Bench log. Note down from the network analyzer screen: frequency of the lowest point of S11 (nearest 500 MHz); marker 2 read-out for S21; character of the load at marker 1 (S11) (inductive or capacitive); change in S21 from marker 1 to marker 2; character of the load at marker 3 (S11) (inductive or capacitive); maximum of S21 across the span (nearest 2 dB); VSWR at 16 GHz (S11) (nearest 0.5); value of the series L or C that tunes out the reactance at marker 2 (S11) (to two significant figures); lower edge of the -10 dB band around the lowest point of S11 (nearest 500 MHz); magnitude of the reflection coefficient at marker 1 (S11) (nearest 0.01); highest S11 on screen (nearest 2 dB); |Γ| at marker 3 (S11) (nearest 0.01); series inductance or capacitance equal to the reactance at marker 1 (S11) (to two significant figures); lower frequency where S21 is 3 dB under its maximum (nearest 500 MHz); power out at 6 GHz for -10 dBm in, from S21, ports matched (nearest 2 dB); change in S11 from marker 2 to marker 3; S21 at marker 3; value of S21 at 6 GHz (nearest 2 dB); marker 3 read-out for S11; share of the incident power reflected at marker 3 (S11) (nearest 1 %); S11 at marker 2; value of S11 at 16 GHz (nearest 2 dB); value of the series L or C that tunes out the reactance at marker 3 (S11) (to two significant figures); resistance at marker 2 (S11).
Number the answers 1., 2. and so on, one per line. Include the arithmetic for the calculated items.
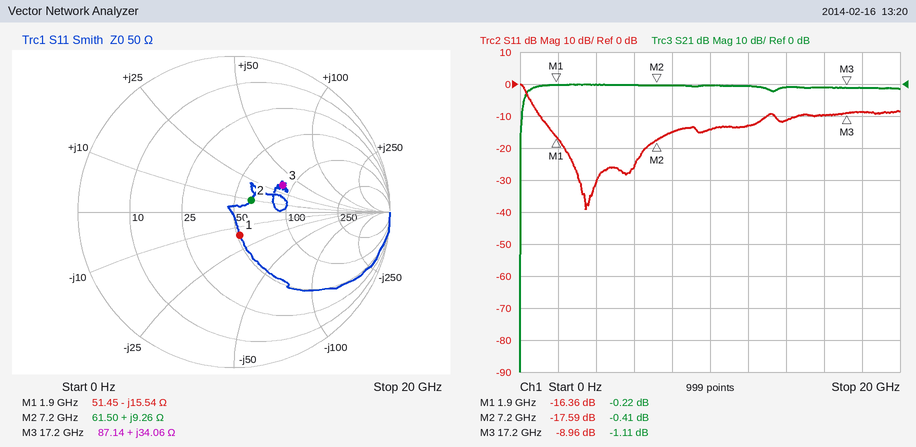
1. 3.5 GHz
2. -0.41 dB
3. capacitive
4. -0.41 − (-0.22) = -0.19 dB
5. inductive
6. 0 dB
7. |Γ| = 10^(-10/20) = 0.3162; VSWR = (1 + 0.3162)/(1 − 0.3162) ≈ 1.92, so 2.0 to the nearest 0.5
8. C = 1/(2π × 7.2 GHz × 9.26 Ω) ≈ 2.4 pF
9. 1.0 GHz
10. 0.15
11. 0 dB
12. 0.36
13. C = 1/(2π × 1.9 GHz × 15.54 Ω) ≈ 5.4 pF
14. 500 MHz
15. -10 dBm + (0 dB) = -10 dBm
16. -8.96 − (-17.59) = 8.63 dB
17. -1.11 dB
18. 0 dB
19. -8.96 dB
20. 10^(-8.96/10) ≈ 13 %
21. -17.59 dB
22. -10 dB
23. C = 1/(2π × 17.2 GHz × 34.06 Ω) ≈ 272 fF, so 270 fF to two significant figures
24. 61.50 Ω
